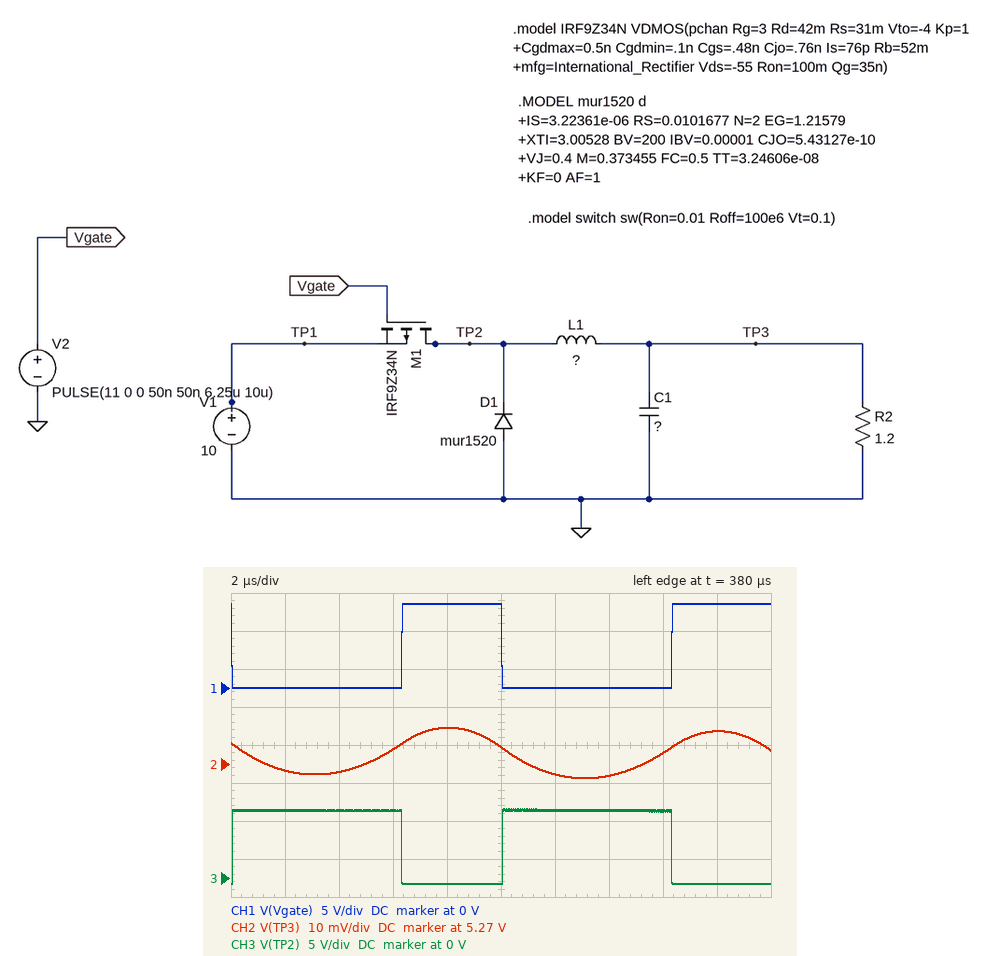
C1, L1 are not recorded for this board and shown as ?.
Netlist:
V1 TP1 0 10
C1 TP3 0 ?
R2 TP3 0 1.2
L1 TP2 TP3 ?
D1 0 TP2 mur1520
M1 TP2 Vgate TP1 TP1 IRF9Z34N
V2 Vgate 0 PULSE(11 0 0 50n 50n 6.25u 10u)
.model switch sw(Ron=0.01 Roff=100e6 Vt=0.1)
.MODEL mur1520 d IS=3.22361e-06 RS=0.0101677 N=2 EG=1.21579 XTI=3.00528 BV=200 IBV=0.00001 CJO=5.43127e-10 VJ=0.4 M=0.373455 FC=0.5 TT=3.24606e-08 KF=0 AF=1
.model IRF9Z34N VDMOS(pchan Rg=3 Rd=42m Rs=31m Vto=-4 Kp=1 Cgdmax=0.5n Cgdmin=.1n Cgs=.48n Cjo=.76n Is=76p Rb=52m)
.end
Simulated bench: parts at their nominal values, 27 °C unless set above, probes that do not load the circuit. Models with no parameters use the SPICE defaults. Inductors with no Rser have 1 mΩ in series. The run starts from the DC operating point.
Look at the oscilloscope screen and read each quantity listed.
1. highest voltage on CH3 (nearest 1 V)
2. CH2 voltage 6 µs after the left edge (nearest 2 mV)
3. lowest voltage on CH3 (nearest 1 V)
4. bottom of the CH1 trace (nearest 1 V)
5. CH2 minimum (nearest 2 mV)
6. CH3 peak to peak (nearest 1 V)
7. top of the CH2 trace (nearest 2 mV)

9 V
5.274 V
-1 V
0 V
5.266 V
10 V
5.280 V
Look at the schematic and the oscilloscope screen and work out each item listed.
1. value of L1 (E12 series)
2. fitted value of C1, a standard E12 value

100 µH
22 µF
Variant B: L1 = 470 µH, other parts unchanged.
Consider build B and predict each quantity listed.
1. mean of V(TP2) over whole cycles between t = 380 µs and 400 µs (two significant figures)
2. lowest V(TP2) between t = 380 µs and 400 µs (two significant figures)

5.5 V
-750 mV
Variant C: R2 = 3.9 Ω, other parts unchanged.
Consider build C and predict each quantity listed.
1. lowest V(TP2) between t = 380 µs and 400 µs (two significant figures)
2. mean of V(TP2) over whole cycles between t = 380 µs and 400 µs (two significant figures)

-700 mV
5.8 V
